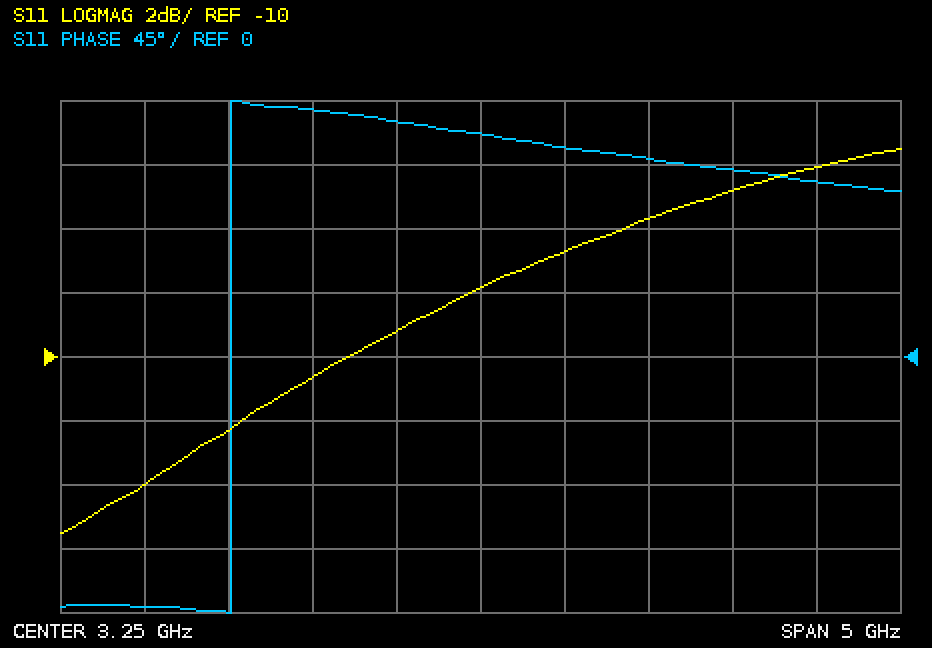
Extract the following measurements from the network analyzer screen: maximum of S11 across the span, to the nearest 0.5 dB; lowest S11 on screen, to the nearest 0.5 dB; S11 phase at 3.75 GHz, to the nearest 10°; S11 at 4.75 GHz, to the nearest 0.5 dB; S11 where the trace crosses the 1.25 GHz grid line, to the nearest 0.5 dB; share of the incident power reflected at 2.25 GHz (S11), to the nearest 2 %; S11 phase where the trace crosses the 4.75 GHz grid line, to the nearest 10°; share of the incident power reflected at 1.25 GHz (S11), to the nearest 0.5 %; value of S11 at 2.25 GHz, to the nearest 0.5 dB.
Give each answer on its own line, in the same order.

-3.5 dB
-15.5 dB
150°
-5.0 dB
-14.0 dB
8 %
130°
4.0 %
-10.5 dB
